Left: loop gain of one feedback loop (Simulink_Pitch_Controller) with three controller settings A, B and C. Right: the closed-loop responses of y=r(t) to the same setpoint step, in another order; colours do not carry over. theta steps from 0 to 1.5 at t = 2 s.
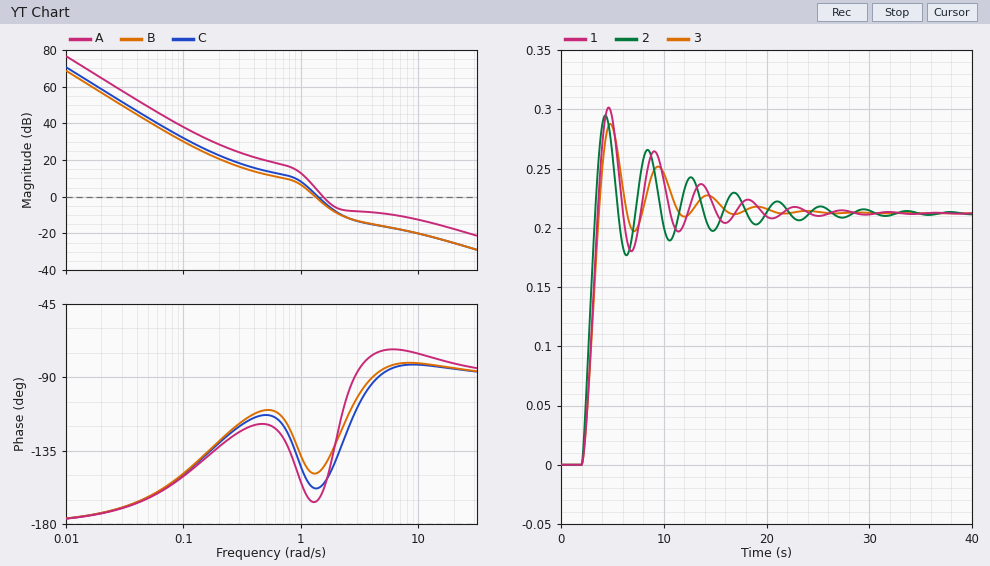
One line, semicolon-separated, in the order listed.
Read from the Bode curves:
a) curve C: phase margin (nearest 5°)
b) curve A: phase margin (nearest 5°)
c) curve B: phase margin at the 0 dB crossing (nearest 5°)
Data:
20°; 20°; 30°
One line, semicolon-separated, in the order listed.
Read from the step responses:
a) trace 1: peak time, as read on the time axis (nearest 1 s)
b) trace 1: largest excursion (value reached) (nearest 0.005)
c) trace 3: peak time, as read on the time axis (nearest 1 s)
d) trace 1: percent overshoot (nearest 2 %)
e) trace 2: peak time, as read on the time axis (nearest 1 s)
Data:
5 s; 0.300; 5 s; 42 %; 4 s
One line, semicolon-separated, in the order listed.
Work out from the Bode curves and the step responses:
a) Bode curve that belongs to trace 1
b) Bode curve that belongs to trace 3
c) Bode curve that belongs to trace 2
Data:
C; B; A
